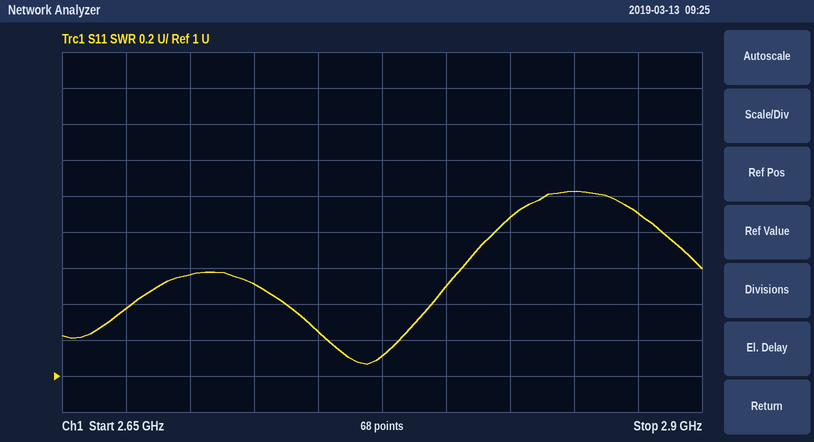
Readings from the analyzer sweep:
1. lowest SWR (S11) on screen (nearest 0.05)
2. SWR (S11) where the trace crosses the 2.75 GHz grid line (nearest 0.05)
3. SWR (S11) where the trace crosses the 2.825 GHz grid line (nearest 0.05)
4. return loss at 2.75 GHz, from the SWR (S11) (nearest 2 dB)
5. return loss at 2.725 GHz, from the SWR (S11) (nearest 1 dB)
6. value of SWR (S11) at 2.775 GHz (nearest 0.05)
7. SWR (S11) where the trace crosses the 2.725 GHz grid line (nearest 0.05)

1.05
1.25
1.90
20 dB
14 dB
1.10
1.50
